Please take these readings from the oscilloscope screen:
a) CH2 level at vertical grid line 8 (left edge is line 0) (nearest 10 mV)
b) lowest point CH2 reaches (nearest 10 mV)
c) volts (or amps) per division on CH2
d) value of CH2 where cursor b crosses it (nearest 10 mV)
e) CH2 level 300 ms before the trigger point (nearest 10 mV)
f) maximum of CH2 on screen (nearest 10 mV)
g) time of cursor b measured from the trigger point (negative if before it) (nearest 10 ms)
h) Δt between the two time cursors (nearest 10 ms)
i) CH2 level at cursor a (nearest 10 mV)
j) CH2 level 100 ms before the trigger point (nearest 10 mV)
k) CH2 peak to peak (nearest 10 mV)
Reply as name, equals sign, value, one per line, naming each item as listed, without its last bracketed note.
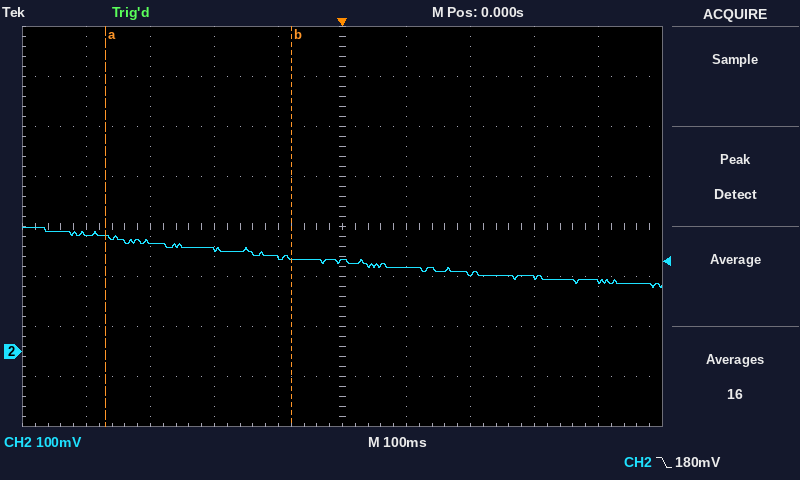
CH2 level at vertical grid line 8 (left edge is line 0) = 150 mV
lowest point CH2 reaches = 130 mV
volts (or amps) per division on CH2 = 100 mV
value of CH2 where cursor b crosses it = 190 mV
CH2 level 300 ms before the trigger point = 220 mV
maximum of CH2 on screen = 250 mV
time of cursor b measured from the trigger point (negative if before it) = -80 ms
Δt between the two time cursors = 290 ms
CH2 level at cursor a = 230 mV
CH2 level 100 ms before the trigger point = 190 mV
CH2 peak to peak = 120 mV
